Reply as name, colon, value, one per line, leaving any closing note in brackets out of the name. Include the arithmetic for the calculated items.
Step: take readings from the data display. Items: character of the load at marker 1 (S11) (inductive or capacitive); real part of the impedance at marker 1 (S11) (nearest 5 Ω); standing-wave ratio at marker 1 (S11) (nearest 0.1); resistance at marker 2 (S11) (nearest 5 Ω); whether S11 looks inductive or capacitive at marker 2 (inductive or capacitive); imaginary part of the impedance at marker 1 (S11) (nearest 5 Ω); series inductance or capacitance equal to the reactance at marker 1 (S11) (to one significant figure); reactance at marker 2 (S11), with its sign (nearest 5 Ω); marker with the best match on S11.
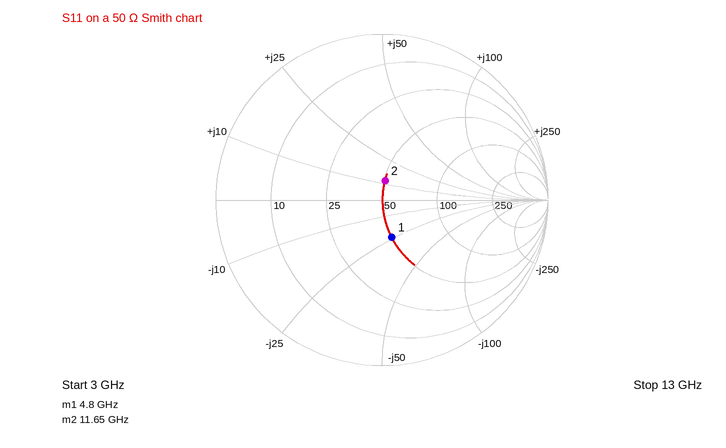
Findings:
character of the load at marker 1 (S11): capacitive
real part of the impedance at marker 1 (S11): 50 Ω
standing-wave ratio at marker 1 (S11): 1.6
resistance at marker 2 (S11): 50 Ω
whether S11 looks inductive or capacitive at marker 2: inductive
imaginary part of the impedance at marker 1 (S11): -25 Ω
series inductance or capacitance equal to the reactance at marker 1 (S11): C = 1/(2π × 4.8 GHz × 25 Ω) ≈ 1 pF
reactance at marker 2 (S11), with its sign: +10 Ω
marker with the best match on S11: marker 2
